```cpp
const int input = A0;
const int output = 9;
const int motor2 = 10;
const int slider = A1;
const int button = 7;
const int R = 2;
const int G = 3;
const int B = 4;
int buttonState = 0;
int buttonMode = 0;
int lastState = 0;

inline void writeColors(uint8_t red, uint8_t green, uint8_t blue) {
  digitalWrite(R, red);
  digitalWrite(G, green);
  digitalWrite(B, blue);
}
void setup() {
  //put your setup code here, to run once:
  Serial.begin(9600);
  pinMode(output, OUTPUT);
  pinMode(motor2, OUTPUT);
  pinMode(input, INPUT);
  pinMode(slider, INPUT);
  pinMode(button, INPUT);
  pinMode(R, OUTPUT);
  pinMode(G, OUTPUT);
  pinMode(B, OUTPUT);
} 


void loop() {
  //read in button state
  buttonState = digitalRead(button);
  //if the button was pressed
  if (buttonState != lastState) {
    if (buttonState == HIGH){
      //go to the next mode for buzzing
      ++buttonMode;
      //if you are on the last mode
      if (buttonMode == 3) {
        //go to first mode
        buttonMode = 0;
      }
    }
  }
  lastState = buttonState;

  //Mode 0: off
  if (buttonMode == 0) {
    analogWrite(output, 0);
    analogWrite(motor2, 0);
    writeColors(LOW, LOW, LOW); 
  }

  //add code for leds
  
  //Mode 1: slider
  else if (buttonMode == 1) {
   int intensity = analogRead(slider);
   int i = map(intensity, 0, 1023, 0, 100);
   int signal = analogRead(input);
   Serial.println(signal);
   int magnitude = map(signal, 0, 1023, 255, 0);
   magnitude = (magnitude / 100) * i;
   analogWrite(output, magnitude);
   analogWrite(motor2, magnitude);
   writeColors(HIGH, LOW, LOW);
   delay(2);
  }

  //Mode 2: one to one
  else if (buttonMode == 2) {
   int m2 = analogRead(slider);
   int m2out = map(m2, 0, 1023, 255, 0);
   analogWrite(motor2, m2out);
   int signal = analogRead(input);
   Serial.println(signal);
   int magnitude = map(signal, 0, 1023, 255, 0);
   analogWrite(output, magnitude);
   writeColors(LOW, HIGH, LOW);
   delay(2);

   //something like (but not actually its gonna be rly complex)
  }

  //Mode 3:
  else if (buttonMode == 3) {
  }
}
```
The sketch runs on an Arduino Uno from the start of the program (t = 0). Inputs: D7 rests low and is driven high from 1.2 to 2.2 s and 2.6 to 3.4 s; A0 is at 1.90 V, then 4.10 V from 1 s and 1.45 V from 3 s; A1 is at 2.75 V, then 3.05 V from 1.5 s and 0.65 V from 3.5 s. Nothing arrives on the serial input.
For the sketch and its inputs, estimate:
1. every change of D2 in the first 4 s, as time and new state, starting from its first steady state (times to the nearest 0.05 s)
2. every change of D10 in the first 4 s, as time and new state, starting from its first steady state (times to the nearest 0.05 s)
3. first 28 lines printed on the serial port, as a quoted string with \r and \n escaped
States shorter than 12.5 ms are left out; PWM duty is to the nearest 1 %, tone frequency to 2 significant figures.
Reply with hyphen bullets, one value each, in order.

- 0 s low; 1.2 s high; 2.6 s low
- 0 s low; 2.6 s PWM 39 %; 3.5 s PWM 87 %
- "839\r\n839\r\n839\r\n839\r\n839\r\n839\r\n839\r\n839\r\n839\r\n839\r\n839\r\n839\r\n839\r\n839\r\n839\r\n839\r\n839\r\n839\r\n839\r\n839\r\n839\r\n839\r\n839\r\n839\r\n839\r\n839\r\n839\r\n839\r\n"
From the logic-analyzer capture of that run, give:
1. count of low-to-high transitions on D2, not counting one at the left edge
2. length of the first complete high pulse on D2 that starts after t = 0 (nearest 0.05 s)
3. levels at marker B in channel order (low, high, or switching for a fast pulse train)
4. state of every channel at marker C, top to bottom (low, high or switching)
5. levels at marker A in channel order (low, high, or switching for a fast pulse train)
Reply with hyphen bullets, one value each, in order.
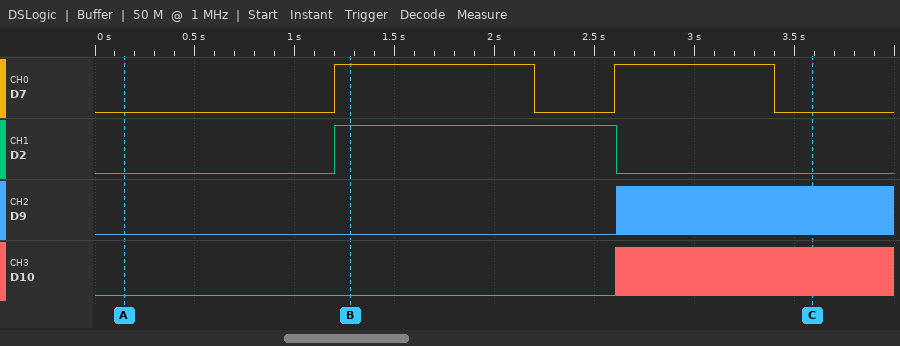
- 1
- 1.40 s
- D7 high, D2 high, D9 low, D10 low
- D7 low, D2 low, D9 switching, D10 switching
- D7 low, D2 low, D9 low, D10 low
